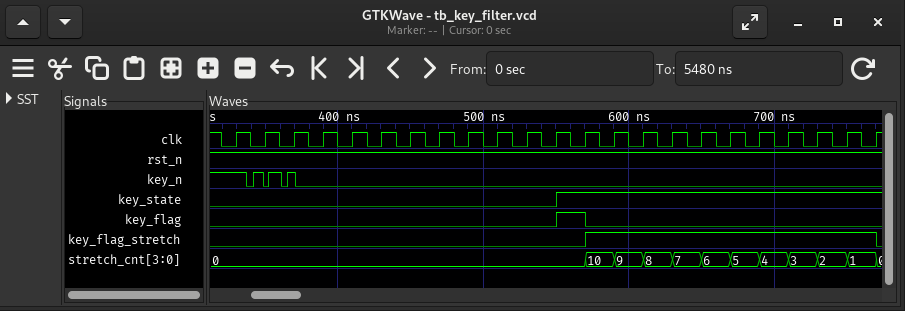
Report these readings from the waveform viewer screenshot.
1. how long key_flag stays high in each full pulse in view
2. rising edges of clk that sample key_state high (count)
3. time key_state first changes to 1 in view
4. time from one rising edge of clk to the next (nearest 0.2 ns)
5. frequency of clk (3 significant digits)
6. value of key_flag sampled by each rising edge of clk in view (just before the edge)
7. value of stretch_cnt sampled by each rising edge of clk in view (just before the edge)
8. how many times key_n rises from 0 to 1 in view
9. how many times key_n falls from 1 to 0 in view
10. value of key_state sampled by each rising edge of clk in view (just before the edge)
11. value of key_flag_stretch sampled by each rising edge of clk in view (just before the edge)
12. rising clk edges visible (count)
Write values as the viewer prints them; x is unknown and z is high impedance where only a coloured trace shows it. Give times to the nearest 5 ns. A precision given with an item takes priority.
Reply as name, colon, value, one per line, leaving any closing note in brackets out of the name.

how long key_flag stays high in each full pulse in view: 20 ns
rising edges of clk that sample key_state high: 11
time key_state first changes to 1 in view: 550 ns
time from one rising edge of clk to the next: 20 ns
frequency of clk: 50.0 MHz
value of key_flag sampled by each rising edge of clk in view: 0 0 0 0 0 0 0 0 0 0 0 0 1 0 0 0 0 0 0 0 0 0 0
value of stretch_cnt sampled by each rising edge of clk in view: 0, 0, 0, 0, 0, 0, 0, 0, 0, 0, 0, 0, 0, 10, 9, 8, 7, 6, 5, 4, 3, 2, 1
how many times key_n rises from 0 to 1 in view: 3
how many times key_n falls from 1 to 0 in view: 4
value of key_state sampled by each rising edge of clk in view: 0 0 0 0 0 0 0 0 0 0 0 0 1 1 1 1 1 1 1 1 1 1 1
value of key_flag_stretch sampled by each rising edge of clk in view: 0 0 0 0 0 0 0 0 0 0 0 0 0 1 1 1 1 1 1 1 1 1 1
rising clk edges visible: 23
